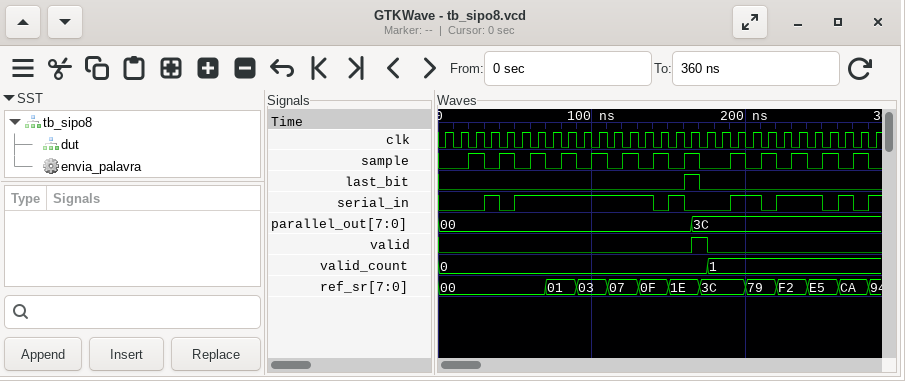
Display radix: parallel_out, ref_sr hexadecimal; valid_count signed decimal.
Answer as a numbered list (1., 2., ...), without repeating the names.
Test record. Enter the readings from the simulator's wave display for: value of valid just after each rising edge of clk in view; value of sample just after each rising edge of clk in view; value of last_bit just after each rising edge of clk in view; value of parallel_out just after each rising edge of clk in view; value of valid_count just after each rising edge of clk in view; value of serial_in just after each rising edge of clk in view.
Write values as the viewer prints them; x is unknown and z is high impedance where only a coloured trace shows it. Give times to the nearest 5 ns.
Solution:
1. 0 0 0 0 0 0 0 0 0 0 0 0 0 0 0 0 1 0 0 0 0 0 0 0 0 0 0 0 0
2. 0 0 1 0 1 0 1 0 1 0 1 0 1 0 1 0 1 0 0 1 0 1 0 1 0 1 0 1 0
3. 0 0 0 0 0 0 0 0 0 0 0 0 0 0 0 0 1 0 0 0 0 0 0 0 0 0 0 0 0
4. 00, 00, 00, 00, 00, 00, 00, 00, 00, 00, 00, 00, 00, 00, 00, 00, 3C, 3C, 3C, 3C, 3C, 3C, 3C, 3C, 3C, 3C, 3C, 3C, 3C
5. 0, 0, 0, 0, 0, 0, 0, 0, 0, 0, 0, 0, 0, 0, 0, 0, 0, 1, 1, 1, 1, 1, 1, 1, 1, 1, 1, 1, 1
6. 0 0 0 1 0 1 1 1 1 1 1 1 1 1 0 1 0 0 0 1 1 0 1 1 1 0 1 0 1
